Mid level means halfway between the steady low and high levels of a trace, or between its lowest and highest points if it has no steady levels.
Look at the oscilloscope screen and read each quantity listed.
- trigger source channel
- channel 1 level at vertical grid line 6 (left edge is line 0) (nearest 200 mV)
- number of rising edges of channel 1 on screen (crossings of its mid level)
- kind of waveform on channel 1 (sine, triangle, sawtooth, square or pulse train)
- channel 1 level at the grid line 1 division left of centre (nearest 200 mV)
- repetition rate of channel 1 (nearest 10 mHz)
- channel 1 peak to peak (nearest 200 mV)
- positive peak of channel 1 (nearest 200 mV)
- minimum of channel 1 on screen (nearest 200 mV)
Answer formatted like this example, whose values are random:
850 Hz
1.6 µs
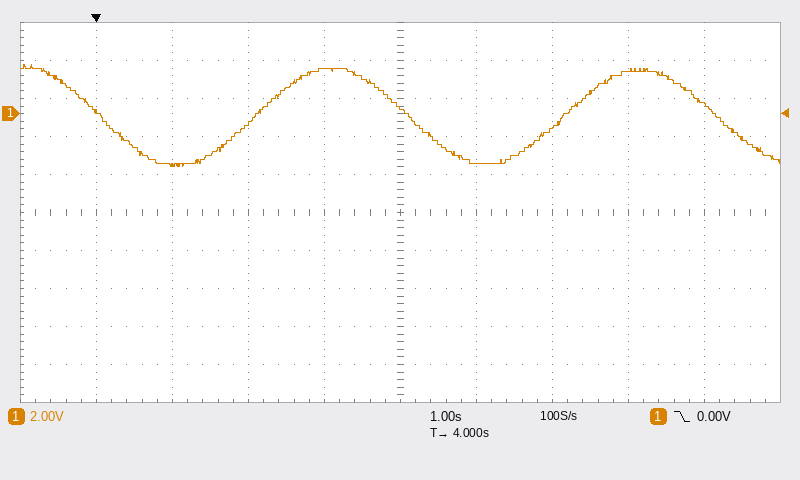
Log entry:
channel 1
-2.6 V
2
sine
2.4 V
250 mHz
5.4 V
2.6 V
-2.8 V
